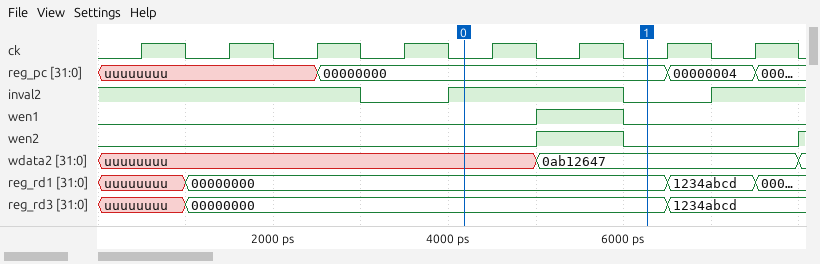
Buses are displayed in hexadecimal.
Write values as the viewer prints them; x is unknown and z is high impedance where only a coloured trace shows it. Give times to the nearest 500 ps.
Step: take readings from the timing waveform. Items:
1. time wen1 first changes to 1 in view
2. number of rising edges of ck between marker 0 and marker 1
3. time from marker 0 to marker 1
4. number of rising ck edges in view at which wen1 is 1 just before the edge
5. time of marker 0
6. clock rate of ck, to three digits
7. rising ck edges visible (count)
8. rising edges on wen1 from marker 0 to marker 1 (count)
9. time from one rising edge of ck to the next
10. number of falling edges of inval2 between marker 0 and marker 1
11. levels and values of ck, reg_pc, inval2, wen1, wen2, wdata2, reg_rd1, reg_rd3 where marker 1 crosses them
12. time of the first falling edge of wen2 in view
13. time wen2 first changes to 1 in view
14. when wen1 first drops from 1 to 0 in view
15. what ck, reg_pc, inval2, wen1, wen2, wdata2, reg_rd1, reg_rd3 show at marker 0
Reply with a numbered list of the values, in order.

1. 5000 ps
2. 2
3. 2000 ps
4. 1
5. 4000 ps
6. 1.00 GHz
7. 8
8. 1
9. 1000 ps
10. 1
11. ck=0, reg_pc=00000000, inval2=0, wen1=0, wen2=0, wdata2=0ab12647, reg_rd1=00000000, reg_rd3=00000000
12. 6000 ps
13. 5000 ps
14. 6000 ps
15. ck=0, reg_pc=00000000, inval2=1, wen1=0, wen2=0, wdata2=uuuuuuuu, reg_rd1=00000000, reg_rd3=00000000
